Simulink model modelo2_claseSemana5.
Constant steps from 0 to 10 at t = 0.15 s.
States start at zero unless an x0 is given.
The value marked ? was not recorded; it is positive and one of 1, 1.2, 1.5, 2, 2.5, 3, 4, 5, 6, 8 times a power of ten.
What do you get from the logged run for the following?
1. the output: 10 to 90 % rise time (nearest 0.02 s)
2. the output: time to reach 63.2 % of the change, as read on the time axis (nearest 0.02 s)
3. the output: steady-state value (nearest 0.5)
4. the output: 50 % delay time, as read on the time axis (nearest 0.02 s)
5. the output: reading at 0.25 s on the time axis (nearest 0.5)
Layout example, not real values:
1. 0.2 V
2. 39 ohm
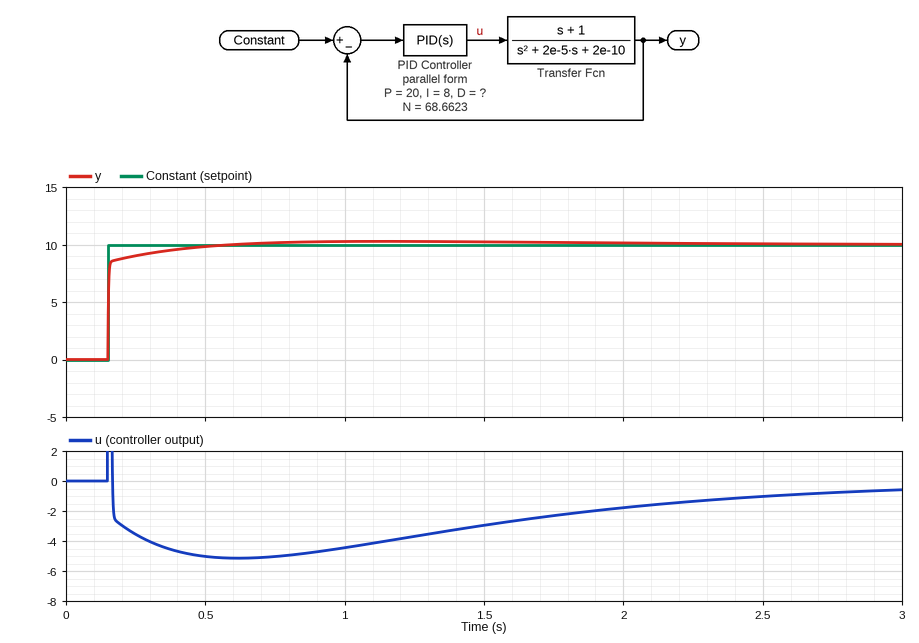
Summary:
1. 0.10 s
2. 0.16 s
3. 10.0
4. 0.16 s
5. 9.0
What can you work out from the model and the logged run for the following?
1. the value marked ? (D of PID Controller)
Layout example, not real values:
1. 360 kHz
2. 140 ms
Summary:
1. 5
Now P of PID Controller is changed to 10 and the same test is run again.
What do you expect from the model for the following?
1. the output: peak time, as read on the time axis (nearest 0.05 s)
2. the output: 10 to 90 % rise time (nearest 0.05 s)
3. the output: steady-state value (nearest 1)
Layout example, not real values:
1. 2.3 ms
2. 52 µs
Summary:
1. 1.50 s
2. 0.15 s
3. 10
